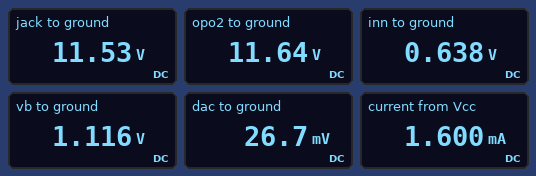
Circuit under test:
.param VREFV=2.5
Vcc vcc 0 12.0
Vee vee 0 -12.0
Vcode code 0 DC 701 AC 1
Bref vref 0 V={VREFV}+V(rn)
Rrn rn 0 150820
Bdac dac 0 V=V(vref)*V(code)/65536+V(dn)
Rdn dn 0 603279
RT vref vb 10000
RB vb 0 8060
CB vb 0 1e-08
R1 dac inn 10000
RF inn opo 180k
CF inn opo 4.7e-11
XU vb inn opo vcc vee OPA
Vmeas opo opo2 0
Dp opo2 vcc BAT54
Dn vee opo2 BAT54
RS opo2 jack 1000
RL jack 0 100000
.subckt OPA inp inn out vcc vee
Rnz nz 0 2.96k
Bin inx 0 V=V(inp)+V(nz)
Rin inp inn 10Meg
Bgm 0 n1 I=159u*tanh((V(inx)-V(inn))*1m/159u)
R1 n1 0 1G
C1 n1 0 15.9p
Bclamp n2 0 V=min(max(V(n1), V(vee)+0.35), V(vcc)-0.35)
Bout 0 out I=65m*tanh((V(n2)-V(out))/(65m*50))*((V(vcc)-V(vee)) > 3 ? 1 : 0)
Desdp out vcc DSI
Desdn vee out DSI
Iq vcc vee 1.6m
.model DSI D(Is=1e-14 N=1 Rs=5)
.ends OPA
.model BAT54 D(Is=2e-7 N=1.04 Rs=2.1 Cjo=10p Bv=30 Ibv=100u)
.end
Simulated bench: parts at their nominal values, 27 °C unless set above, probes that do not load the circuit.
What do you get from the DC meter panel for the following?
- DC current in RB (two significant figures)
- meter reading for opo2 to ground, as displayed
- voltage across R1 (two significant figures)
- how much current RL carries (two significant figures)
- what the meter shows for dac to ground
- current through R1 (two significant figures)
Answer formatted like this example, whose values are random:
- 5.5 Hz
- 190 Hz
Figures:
- 140 µA
- 11.64 V
- 610 mV
- 120 µA
- 26.7 mV
- 61 µA
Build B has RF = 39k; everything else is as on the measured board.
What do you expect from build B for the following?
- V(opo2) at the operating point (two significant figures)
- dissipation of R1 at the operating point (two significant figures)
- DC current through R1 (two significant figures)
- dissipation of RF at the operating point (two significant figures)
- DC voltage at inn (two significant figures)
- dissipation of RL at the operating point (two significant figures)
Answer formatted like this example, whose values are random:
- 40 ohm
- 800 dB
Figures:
- 5.4 V
- 120 µW
- 110 µA
- 460 µW
- 1.1 V
- 280 µW
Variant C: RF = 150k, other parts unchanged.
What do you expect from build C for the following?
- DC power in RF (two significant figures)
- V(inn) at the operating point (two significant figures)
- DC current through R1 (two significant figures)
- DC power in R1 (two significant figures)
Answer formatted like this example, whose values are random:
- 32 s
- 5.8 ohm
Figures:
- 790 µW
- 750 mV
- 73 µA
- 53 µW
